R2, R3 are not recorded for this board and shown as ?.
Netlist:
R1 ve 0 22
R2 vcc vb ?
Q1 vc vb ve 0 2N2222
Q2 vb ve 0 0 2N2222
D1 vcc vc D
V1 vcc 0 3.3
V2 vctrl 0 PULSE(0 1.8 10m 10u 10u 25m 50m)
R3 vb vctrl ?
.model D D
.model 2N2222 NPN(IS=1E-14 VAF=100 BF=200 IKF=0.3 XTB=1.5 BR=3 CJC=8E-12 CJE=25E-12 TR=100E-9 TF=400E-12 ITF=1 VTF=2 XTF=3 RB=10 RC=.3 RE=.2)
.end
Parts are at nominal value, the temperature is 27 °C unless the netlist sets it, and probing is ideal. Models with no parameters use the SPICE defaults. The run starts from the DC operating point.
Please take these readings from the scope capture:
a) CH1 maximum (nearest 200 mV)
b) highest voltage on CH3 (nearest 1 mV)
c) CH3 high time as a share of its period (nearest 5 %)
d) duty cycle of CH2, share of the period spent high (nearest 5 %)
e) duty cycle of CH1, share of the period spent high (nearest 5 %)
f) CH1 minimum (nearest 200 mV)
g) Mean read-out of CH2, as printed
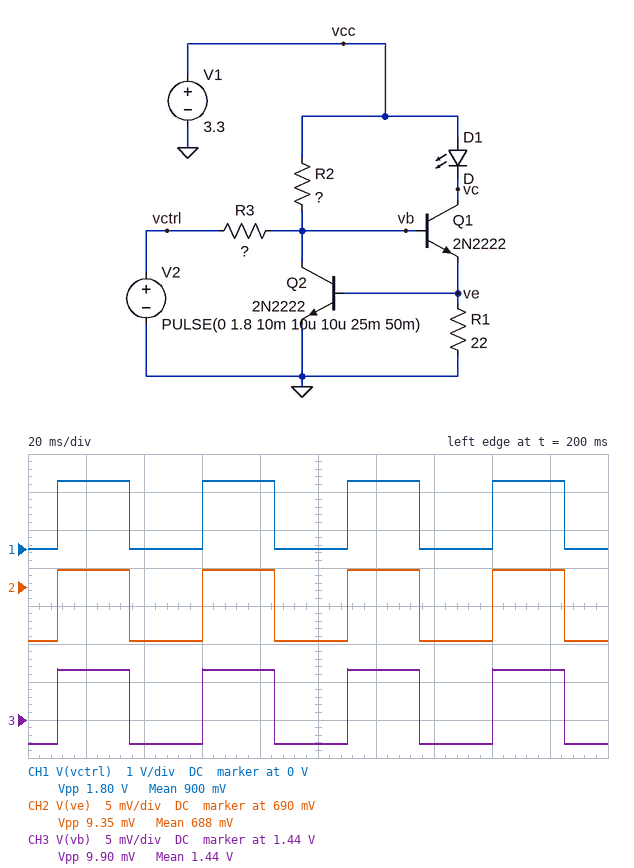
1.8 V
1.447 V
50 %
50 %
50 %
0 V
688 mV
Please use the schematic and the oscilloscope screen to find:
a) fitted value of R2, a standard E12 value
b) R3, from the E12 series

470 Ω
1.5 kΩ
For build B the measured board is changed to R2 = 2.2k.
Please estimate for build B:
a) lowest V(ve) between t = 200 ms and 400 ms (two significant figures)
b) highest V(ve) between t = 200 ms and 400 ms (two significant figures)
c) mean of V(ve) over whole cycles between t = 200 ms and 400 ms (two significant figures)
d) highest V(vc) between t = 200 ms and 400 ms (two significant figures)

490 mV
650 mV
570 mV
2.6 V
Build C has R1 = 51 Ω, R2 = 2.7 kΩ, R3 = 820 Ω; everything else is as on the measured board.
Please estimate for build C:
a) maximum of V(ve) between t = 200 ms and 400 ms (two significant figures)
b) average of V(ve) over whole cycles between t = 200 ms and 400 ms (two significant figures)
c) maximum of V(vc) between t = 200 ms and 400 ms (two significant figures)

660 mV
380 mV
2.6 V
